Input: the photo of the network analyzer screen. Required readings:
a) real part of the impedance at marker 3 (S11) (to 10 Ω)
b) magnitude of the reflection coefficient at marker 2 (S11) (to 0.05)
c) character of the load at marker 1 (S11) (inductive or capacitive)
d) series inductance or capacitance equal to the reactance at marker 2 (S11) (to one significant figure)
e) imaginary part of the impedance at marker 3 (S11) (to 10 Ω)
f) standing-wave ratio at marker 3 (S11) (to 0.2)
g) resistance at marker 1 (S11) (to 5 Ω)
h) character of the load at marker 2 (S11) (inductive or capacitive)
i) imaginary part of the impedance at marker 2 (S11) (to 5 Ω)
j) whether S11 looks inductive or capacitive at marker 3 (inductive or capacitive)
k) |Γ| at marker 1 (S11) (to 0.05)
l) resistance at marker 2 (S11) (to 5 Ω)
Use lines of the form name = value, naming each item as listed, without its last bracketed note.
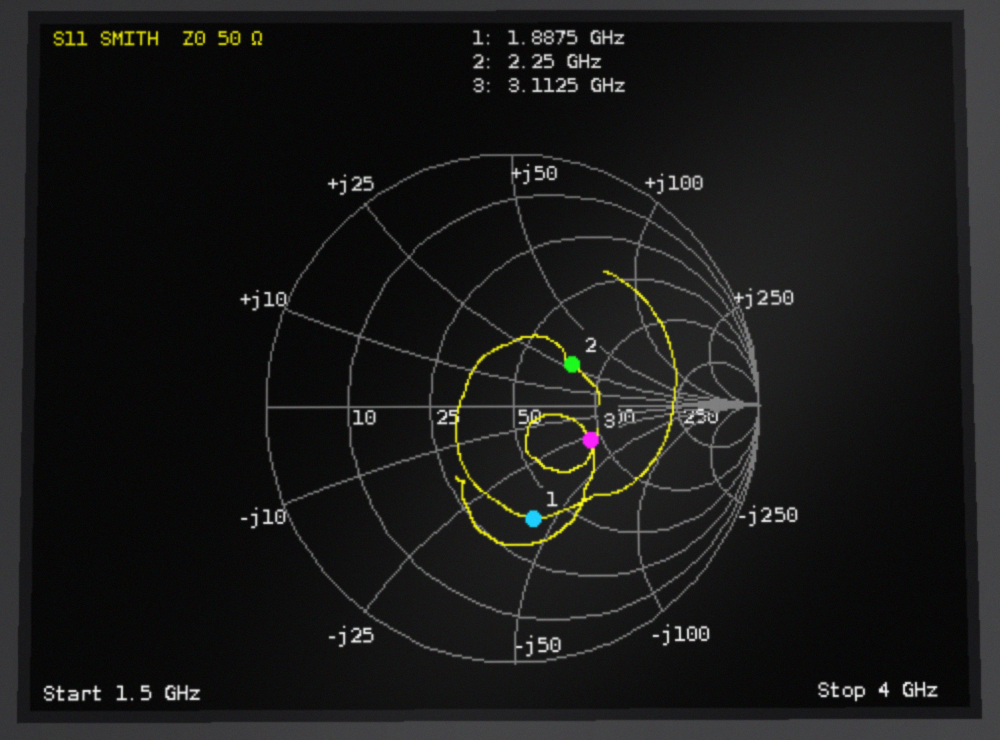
real part of the impedance at marker 3 (S11) = 90 Ω
magnitude of the reflection coefficient at marker 2 (S11) = 0.30
character of the load at marker 1 (S11) = capacitive
series inductance or capacitance equal to the reactance at marker 2 (S11) = 2 nH
imaginary part of the impedance at marker 3 (S11) = -30 Ω
standing-wave ratio at marker 3 (S11) = 2.0
resistance at marker 1 (S11) = 40 Ω
character of the load at marker 2 (S11) = inductive
imaginary part of the impedance at marker 2 (S11) = +25 Ω
whether S11 looks inductive or capacitive at marker 3 = capacitive
|Γ| at marker 1 (S11) = 0.45
resistance at marker 2 (S11) = 75 Ω
